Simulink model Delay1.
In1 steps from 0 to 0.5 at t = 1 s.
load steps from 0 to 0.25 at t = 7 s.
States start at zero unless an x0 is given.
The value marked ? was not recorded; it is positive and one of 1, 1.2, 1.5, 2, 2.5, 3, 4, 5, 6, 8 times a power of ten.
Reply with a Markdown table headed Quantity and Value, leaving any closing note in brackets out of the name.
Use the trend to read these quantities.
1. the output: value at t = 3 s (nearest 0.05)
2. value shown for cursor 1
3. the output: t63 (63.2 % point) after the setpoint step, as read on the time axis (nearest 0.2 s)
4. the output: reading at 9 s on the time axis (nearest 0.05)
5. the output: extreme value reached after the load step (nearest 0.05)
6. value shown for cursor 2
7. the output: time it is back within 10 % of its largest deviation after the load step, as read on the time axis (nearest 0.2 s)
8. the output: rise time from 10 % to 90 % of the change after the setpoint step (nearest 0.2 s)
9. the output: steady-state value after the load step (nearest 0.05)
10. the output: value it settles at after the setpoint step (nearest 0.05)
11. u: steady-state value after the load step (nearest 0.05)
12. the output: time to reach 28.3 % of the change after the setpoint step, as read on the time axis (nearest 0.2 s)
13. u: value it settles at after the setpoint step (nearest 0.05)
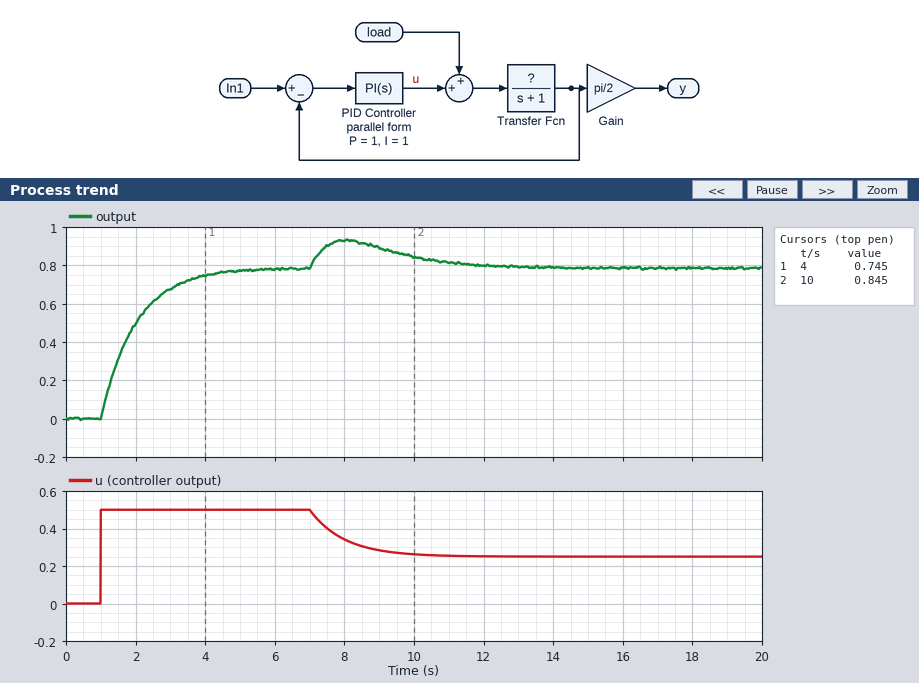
| Quantity | Value |
|---|---|
| the output: value at t = 3 s | 0.70 |
| value shown for cursor 1 | 0.745 |
| the output: t63 (63.2 % point) after the setpoint step, as read on the time axis | 2.0 s |
| the output: reading at 9 s on the time axis | 0.90 |
| the output: extreme value reached after the load step | 0.95 |
| value shown for cursor 2 | 0.845 |
| the output: time it is back within 10 % of its largest deviation after the load step, as read on the time axis | 11.8 s |
| the output: rise time from 10 % to 90 % of the change after the setpoint step | 2.2 s |
| the output: steady-state value after the load step | 0.80 |
| the output: value it settles at after the setpoint step | 0.80 |
| u: steady-state value after the load step | 0.25 |
| the output: time to reach 28.3 % of the change after the setpoint step, as read on the time axis | 1.4 s |
| u: value it settles at after the setpoint step | 0.50 |
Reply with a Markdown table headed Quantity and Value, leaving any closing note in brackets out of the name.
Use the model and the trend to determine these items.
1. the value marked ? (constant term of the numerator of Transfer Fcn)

| Quantity | Value |
|---|---|
| the value marked ? | 1 |
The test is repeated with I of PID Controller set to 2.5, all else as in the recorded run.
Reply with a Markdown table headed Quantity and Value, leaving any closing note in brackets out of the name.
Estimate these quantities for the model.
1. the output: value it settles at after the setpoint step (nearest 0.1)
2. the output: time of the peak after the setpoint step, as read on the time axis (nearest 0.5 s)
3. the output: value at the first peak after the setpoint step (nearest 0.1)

| Quantity | Value |
|---|---|
| the output: value it settles at after the setpoint step | 0.8 |
| the output: time of the peak after the setpoint step, as read on the time axis | 3.0 s |
| the output: value at the first peak after the setpoint step | 0.9 |
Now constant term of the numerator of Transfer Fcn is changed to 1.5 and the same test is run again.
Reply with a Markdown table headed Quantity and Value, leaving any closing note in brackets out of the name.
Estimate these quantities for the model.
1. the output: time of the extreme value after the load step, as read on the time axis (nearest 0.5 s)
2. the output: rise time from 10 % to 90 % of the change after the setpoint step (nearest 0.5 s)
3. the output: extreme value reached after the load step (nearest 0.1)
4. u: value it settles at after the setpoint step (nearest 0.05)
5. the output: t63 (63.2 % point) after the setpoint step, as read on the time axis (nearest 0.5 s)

| Quantity | Value |
|---|---|
| the output: time of the extreme value after the load step, as read on the time axis | 8.0 s |
| the output: rise time from 10 % to 90 % of the change after the setpoint step | 1.5 s |
| the output: extreme value reached after the load step | 1.0 |
| u: value it settles at after the setpoint step | 0.35 |
| the output: t63 (63.2 % point) after the setpoint step, as read on the time axis | 1.5 s |
